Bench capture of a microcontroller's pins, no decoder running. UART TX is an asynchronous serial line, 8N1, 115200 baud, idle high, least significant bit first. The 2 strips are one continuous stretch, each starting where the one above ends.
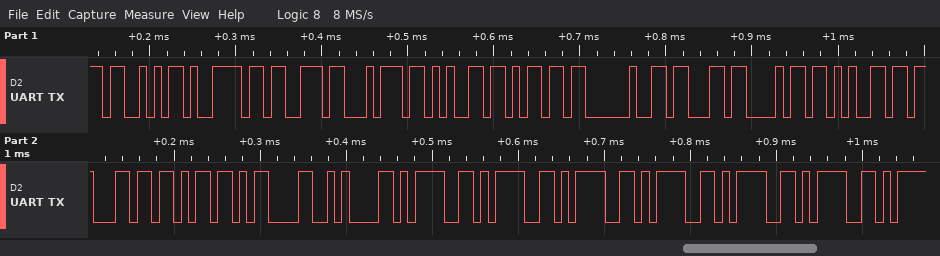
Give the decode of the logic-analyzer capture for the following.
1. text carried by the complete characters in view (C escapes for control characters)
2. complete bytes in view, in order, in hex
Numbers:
"System check\r\n======"
53 79 73 74 65 6D 20 63 68 65 63 6B 0D 0A 3D 3D 3D 3D 3D 3D
